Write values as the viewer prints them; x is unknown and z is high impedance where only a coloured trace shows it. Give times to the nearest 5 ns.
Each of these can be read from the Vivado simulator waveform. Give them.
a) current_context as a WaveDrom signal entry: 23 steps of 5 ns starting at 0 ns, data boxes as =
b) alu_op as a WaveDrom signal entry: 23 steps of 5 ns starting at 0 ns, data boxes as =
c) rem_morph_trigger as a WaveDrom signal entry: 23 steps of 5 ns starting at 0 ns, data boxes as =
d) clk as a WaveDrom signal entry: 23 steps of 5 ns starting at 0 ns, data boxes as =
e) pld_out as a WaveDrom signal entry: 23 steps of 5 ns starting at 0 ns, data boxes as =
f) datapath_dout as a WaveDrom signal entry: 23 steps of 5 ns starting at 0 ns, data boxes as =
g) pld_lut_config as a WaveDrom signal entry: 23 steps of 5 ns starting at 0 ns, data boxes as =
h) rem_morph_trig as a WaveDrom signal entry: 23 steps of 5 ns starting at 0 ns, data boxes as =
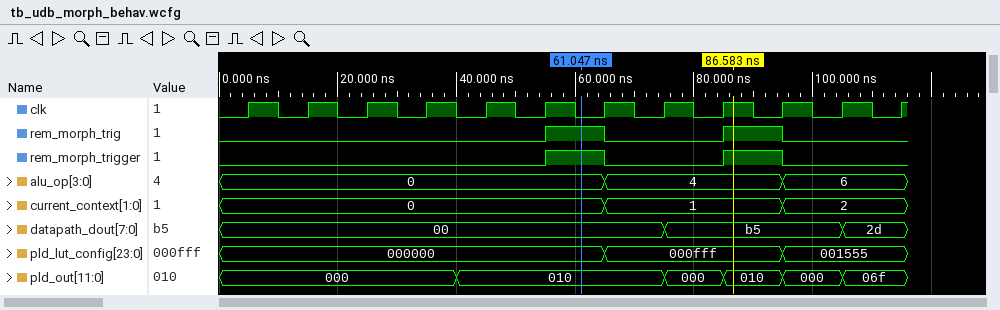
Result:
{name: 'current_context', wave: '=............=.....=...', data: '0 1 2'}
{name: 'alu_op', wave: '=............=.....=...', data: '0 4 6'}
{name: 'rem_morph_trigger', wave: '0..........1.0...1.0...'}
{name: 'clk', wave: '01010101010101010101010'}
{name: 'pld_out', wave: '=.......=......=.=.=.=.', data: '000 010 000 010 000 06f'}
{name: 'datapath_dout', wave: '=..............=.....=.', data: '00 b5 2d'}
{name: 'pld_lut_config', wave: '=............=.....=...', data: '000000 000fff 001555'}
{name: 'rem_morph_trig', wave: '0..........1.0...1.0...'}
